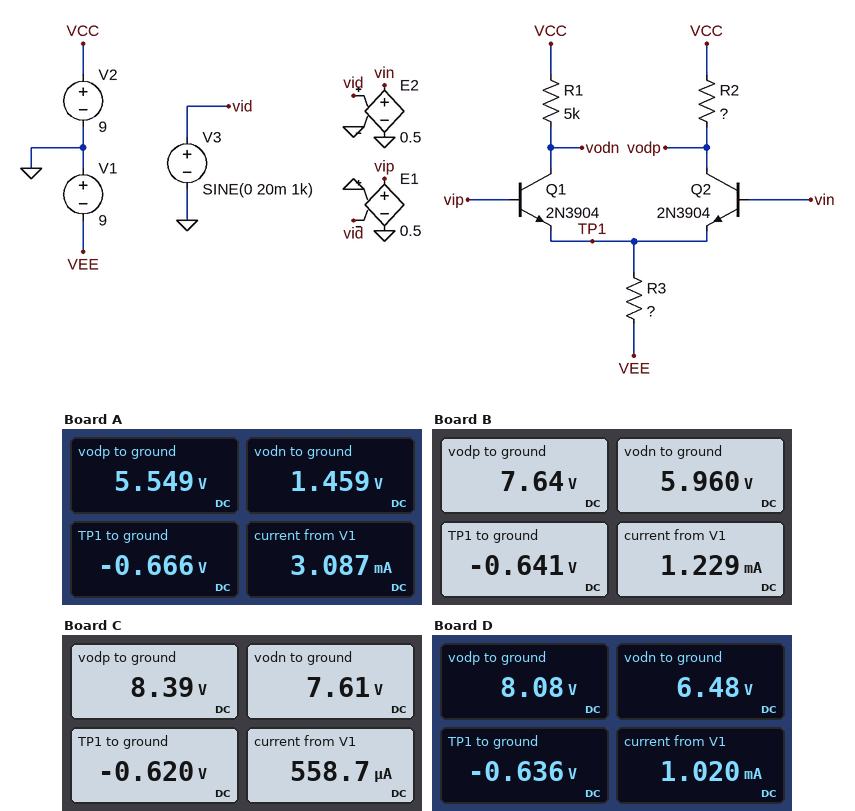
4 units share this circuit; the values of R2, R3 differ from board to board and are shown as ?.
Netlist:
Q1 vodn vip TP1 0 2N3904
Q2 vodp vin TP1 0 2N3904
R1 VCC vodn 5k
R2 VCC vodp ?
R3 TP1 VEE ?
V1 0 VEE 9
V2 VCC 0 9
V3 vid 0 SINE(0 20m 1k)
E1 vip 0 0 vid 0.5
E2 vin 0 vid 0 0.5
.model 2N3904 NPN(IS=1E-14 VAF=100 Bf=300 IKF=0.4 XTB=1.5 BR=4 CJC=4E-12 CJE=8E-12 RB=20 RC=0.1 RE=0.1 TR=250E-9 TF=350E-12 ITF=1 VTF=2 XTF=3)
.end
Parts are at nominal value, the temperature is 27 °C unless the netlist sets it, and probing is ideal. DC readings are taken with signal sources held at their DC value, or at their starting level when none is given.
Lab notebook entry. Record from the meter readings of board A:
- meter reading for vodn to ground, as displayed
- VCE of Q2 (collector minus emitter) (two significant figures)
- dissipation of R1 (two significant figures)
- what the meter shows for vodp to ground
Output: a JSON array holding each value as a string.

["1.459 V", "6.2 V", "11 mW", "5.549 V"]
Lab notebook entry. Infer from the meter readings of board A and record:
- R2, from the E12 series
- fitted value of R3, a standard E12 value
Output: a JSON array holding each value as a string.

["2.2 kΩ", "2.7 kΩ"]
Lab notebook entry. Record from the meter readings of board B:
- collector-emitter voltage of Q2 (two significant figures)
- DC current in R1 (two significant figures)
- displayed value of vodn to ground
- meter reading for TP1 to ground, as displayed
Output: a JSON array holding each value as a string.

["8.3 V", "610 µA", "5.960 V", "-0.641 V"]
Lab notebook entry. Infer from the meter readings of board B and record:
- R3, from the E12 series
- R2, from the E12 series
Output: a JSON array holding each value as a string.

["6.8 kΩ", "2.2 kΩ"]
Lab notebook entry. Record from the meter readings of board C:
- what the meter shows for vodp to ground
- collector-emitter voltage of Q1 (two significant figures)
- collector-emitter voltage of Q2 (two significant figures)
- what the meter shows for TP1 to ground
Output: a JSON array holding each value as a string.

["8.39 V", "8.2 V", "9.0 V", "-0.620 V"]
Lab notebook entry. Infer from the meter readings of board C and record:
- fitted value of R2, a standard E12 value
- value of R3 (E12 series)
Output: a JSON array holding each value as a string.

["2.2 kΩ", "15 kΩ"]
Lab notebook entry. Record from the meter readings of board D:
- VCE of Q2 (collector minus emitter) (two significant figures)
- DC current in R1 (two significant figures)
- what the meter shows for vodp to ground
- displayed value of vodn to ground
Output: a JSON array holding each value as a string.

["8.7 V", "500 µA", "8.08 V", "6.48 V"]
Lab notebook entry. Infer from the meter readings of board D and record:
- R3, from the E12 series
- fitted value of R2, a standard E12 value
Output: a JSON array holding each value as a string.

["8.2 kΩ", "1.8 kΩ"]
